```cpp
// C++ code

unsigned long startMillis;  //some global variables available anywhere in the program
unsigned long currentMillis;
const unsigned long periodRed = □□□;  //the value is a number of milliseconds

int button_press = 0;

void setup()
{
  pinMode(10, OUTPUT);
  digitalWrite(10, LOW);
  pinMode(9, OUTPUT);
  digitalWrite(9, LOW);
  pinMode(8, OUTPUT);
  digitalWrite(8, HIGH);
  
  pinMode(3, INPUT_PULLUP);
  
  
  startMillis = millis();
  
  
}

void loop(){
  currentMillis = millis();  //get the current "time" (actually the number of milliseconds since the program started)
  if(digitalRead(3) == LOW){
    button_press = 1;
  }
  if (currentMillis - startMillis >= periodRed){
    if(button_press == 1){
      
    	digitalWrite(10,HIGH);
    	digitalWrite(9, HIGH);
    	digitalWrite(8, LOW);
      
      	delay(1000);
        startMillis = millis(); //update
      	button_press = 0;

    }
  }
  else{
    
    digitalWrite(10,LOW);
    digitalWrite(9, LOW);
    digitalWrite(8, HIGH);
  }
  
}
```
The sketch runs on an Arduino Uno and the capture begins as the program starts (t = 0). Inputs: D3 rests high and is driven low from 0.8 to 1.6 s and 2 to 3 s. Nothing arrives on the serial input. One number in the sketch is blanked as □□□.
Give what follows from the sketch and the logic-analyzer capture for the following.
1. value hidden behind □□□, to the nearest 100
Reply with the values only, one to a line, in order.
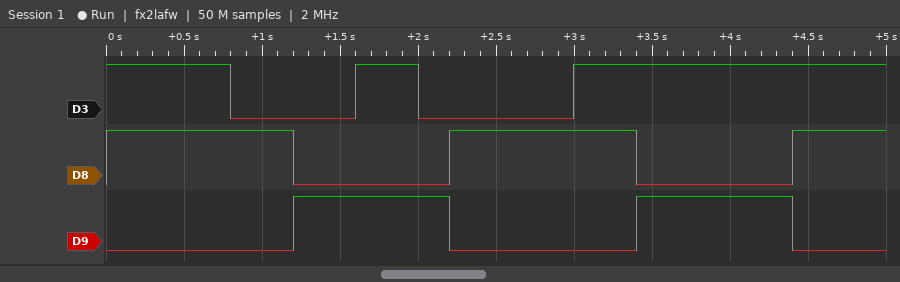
1200
